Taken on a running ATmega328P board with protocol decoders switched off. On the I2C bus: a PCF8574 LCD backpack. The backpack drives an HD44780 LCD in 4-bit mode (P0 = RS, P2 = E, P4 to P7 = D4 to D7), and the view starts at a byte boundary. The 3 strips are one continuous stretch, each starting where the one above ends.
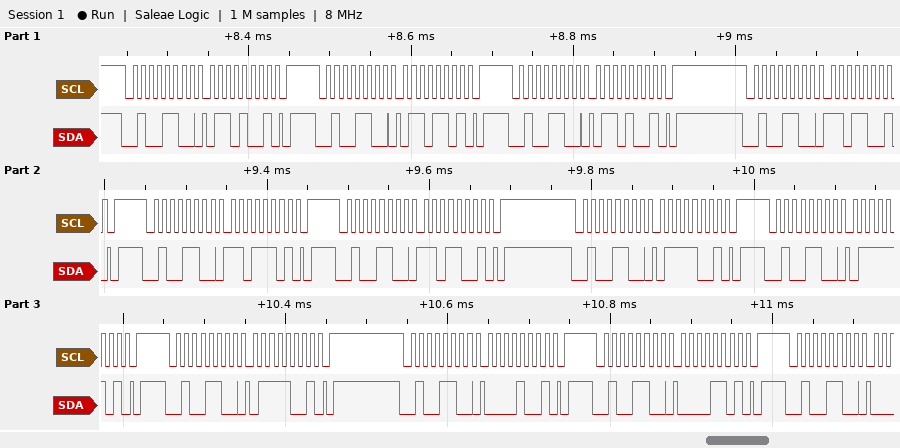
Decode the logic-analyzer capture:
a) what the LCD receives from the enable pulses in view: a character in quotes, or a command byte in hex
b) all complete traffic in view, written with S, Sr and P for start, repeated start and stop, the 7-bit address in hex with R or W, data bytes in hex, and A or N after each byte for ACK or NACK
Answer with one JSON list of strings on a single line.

["'m'", "S 26W A 69 A P S 26W A 6D A P S 26W A 69 A P S 26W A D9 A P S 26W A DD A P S 26W A D9 A P S 26W A 79 A P S 26W A 7D A P S 26W A 79 A P S 26W A 09 A P S 26W A 0D A P S 26W A"]
